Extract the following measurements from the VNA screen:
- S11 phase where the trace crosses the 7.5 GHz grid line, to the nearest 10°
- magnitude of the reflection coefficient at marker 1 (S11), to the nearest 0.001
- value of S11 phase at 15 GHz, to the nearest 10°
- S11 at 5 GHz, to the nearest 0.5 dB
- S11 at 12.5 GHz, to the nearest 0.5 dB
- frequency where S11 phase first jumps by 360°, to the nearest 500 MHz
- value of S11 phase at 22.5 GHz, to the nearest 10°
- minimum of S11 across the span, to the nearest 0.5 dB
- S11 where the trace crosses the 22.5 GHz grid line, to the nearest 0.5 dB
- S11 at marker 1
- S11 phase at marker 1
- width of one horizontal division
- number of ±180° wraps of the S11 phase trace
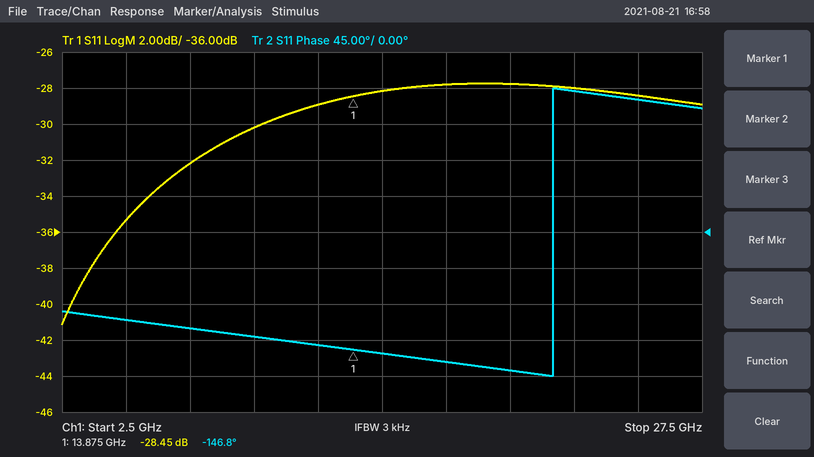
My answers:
-120°
0.038
-150°
-35.5 dB
-29.0 dB
21.5 GHz
180°
-41.0 dB
-28.0 dB
-28.45 dB
-146.8°
2.5 GHz
1
